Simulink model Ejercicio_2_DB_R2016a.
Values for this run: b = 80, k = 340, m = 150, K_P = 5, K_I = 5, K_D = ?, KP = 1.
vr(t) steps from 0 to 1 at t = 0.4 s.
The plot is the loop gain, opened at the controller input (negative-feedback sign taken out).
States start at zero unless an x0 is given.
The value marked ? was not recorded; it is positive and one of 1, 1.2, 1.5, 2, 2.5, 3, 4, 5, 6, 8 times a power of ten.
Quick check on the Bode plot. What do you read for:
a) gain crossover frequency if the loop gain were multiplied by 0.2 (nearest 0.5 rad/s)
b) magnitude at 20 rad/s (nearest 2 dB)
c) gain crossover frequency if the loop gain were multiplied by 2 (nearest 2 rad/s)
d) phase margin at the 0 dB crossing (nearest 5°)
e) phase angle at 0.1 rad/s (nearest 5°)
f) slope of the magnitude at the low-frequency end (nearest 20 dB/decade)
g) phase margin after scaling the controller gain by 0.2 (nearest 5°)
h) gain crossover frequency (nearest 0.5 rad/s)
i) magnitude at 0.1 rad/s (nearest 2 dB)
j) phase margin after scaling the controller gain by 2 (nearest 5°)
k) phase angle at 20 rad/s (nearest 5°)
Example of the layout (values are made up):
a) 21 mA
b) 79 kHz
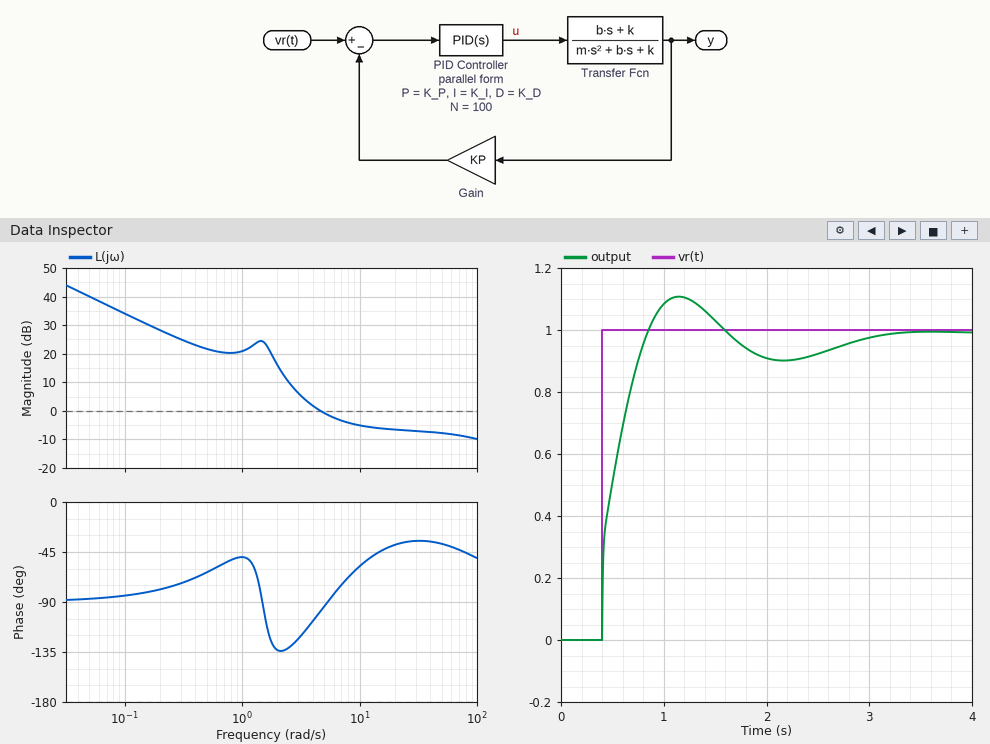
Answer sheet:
a) 2.0 rad/s
b) -6 dB
c) 14 rad/s
d) 80°
e) -85°
f) -20 dB/decade
g) 45°
h) 4.5 rad/s
i) 34 dB
j) 135°
k) -40°
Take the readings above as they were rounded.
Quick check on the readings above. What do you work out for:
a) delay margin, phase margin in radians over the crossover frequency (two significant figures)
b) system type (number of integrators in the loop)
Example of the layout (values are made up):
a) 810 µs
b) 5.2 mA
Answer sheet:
a) 0.31 s
b) 1
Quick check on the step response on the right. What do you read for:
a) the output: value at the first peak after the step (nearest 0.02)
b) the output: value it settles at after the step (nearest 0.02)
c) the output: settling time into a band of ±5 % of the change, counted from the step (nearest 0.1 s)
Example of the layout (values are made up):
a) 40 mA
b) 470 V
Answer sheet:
a) 1.10
b) 1.00
c) 2.3 s
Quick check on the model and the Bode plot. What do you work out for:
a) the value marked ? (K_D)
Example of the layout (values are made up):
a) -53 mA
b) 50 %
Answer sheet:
a) 0.8
